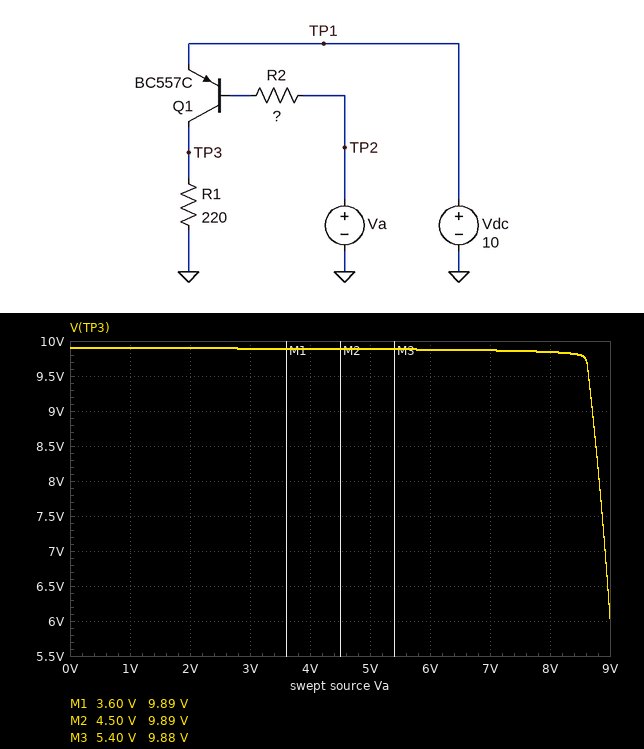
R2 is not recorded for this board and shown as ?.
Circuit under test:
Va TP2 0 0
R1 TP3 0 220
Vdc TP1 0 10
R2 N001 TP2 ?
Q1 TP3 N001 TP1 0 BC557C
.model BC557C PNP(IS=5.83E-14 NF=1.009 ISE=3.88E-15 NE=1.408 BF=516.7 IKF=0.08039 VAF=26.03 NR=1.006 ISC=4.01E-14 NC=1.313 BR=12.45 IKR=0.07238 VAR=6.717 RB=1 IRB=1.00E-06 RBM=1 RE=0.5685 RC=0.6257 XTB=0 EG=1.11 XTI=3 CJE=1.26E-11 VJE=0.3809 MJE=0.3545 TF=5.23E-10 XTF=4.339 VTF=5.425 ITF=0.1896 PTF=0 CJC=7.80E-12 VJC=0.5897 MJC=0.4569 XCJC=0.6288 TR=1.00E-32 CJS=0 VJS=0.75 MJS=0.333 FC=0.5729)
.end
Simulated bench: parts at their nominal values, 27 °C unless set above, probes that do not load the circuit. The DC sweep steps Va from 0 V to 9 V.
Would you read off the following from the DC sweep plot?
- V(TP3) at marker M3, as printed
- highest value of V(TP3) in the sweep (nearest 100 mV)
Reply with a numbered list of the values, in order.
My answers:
1. 9.88 V
2. 9.9 V
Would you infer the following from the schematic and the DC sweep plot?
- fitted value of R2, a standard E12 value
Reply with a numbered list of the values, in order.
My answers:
1. 3.9 kΩ
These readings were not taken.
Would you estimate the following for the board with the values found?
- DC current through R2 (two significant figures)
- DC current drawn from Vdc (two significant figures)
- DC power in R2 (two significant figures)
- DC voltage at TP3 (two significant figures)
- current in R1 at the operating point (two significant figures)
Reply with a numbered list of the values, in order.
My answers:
1. 2.4 mA
2. 47 mA
3. 22 mW
4. 9.9 V
5. 45 mA
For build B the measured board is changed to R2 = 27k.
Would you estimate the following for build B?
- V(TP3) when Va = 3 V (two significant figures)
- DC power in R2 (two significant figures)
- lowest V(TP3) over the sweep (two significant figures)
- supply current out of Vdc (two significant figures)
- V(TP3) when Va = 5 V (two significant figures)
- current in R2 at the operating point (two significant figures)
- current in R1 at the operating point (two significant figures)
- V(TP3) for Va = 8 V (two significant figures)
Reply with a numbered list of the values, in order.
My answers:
1. 9.8 V
2. 3.2 mW
3. 1.5 V
4. 45 mA
5. 9.6 V
6. 340 µA
7. 45 mA
8. 4.6 V
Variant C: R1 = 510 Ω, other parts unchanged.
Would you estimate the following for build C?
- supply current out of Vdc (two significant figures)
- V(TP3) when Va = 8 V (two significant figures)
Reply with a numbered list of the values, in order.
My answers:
1. 22 mA
2. 9.9 V
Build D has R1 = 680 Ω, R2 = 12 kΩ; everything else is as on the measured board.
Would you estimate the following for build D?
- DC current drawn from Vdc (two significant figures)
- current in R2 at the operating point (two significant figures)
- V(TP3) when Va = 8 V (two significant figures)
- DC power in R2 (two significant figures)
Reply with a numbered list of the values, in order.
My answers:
1. 15 mA
2. 770 µA
3. 9.9 V
4. 7.2 mW
